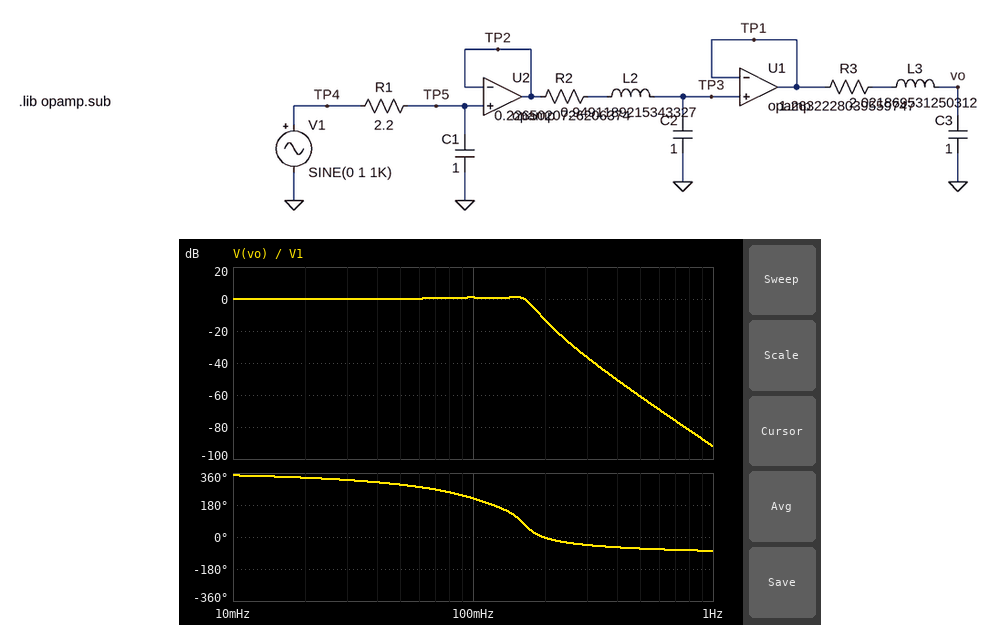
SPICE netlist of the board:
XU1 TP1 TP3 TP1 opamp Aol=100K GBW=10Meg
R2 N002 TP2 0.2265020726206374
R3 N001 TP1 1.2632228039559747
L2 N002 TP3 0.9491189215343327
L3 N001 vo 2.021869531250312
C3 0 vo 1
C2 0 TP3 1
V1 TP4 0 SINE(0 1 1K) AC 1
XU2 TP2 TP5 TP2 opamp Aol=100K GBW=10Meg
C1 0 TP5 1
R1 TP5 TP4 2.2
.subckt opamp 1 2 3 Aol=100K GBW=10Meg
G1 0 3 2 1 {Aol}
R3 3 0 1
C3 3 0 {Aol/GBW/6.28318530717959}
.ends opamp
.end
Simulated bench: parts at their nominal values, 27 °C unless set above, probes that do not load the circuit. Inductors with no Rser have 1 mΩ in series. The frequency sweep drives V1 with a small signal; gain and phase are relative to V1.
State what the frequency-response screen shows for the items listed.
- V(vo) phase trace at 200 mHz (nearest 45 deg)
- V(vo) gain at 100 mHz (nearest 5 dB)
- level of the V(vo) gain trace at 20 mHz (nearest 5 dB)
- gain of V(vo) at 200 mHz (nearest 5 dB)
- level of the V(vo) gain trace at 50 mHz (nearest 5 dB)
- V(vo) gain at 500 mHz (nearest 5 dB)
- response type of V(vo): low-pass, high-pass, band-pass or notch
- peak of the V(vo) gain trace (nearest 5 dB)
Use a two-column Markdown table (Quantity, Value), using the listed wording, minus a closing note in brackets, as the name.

| Quantity | Value |
|---|---|
| V(vo) phase trace at 200 mHz | 0 deg |
| V(vo) gain at 100 mHz | 0 dB |
| level of the V(vo) gain trace at 20 mHz | 0 dB |
| gain of V(vo) at 200 mHz | -15 dB |
| level of the V(vo) gain trace at 50 mHz | 0 dB |
| V(vo) gain at 500 mHz | -60 dB |
| response type of V(vo): low-pass, high-pass, band-pass or notch | low-pass |
| peak of the V(vo) gain trace | 0 dB |
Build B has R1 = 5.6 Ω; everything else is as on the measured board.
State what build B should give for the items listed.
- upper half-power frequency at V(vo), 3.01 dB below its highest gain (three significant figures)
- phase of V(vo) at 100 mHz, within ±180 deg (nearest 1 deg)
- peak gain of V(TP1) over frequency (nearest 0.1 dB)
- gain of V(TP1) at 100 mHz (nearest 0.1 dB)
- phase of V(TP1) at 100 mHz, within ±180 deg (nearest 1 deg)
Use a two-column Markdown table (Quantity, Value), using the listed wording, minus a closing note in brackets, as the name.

| Quantity | Value |
|---|---|
| upper half-power frequency at V(vo), 3.01 dB below its highest gain | 34.0 mHz |
| phase of V(vo) at 100 mHz, within ±180 deg | -163 deg |
| peak gain of V(TP1) over frequency | 0 dB |
| gain of V(TP1) at 100 mHz | -7.4 dB |
| phase of V(TP1) at 100 mHz, within ±180 deg | -87 deg |
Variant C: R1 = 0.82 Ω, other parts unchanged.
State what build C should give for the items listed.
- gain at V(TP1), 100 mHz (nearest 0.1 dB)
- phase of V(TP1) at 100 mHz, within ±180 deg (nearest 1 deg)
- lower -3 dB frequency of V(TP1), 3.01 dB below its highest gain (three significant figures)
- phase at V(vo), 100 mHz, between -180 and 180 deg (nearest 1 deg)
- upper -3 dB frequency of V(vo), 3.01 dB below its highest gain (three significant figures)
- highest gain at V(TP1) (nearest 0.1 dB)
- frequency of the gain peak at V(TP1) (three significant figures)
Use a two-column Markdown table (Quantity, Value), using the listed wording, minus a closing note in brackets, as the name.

| Quantity | Value |
|---|---|
| gain at V(TP1), 100 mHz | 2.8 dB |
| phase of V(TP1) at 100 mHz, within ±180 deg | -40 deg |
| lower -3 dB frequency of V(TP1), 3.01 dB below its highest gain | 138 mHz |
| phase at V(vo), 100 mHz, between -180 and 180 deg | -116 deg |
| upper -3 dB frequency of V(vo), 3.01 dB below its highest gain | 171 mHz |
| highest gain at V(TP1) | 10.4 dB |
| frequency of the gain peak at V(TP1) | 160 mHz |
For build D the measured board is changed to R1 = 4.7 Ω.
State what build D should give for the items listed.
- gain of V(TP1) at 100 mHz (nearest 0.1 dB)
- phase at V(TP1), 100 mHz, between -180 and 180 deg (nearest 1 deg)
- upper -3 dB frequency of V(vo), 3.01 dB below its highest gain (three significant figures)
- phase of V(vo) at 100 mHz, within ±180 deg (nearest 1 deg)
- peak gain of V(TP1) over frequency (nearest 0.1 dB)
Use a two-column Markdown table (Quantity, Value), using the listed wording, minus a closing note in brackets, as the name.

| Quantity | Value |
|---|---|
| gain of V(TP1) at 100 mHz | -6.0 dB |
| phase at V(TP1), 100 mHz, between -180 and 180 deg | -84 deg |
| upper -3 dB frequency of V(vo), 3.01 dB below its highest gain | 46.1 mHz |
| phase of V(vo) at 100 mHz, within ±180 deg | -160 deg |
| peak gain of V(TP1) over frequency | 0 dB |
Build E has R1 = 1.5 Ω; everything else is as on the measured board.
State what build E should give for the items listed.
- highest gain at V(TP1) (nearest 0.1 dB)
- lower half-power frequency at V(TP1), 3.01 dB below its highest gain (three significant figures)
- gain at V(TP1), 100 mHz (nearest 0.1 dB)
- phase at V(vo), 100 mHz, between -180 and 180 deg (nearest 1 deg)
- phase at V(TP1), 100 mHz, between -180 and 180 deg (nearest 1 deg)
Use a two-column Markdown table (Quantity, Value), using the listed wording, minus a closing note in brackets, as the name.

| Quantity | Value |
|---|---|
| highest gain at V(TP1) | 7.5 dB |
| lower half-power frequency at V(TP1), 3.01 dB below its highest gain | 136 mHz |
| gain at V(TP1), 100 mHz | 1.1 dB |
| phase at V(vo), 100 mHz, between -180 and 180 deg | -132 deg |
| phase at V(TP1), 100 mHz, between -180 and 180 deg | -56 deg |
